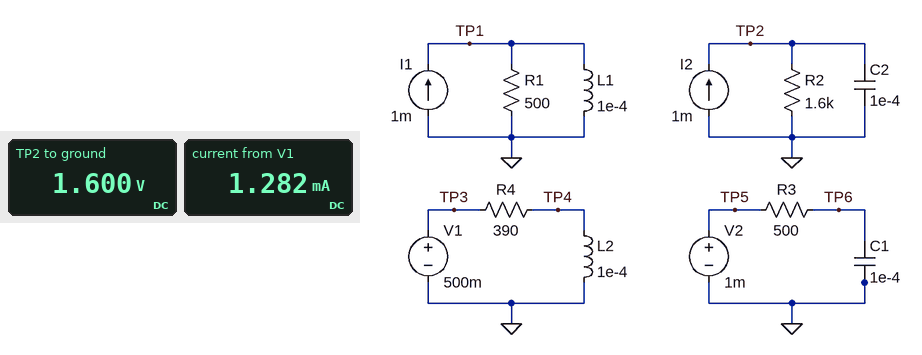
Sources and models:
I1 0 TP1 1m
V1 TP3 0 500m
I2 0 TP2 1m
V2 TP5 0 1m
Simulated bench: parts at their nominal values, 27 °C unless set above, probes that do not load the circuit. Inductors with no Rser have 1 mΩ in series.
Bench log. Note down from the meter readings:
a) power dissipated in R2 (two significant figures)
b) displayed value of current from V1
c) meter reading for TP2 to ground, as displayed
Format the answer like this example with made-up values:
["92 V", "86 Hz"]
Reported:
["1.6 mW", "1.282 mA", "1.600 V"]
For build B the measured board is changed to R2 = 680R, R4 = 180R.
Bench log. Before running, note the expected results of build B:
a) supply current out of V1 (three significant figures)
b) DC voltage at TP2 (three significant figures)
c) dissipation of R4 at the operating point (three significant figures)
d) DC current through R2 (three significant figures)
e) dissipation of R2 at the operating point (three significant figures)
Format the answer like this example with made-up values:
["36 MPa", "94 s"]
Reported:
["2.78 mA", "680 mV", "1.39 mW", "1.00 mA", "680 µW"]
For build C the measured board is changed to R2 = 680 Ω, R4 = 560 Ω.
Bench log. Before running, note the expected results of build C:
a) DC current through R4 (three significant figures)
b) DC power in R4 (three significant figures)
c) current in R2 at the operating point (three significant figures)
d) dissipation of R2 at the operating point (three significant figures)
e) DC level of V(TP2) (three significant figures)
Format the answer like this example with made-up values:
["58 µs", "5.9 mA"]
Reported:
["893 µA", "446 µW", "1.00 mA", "680 µW", "680 mV"]
